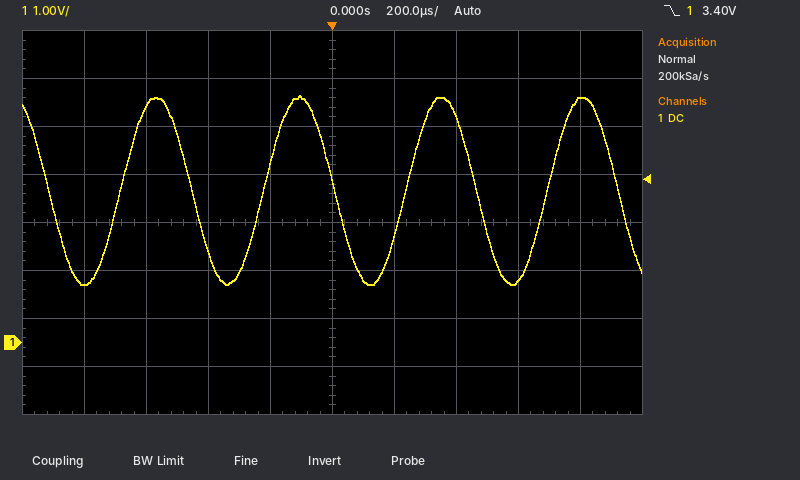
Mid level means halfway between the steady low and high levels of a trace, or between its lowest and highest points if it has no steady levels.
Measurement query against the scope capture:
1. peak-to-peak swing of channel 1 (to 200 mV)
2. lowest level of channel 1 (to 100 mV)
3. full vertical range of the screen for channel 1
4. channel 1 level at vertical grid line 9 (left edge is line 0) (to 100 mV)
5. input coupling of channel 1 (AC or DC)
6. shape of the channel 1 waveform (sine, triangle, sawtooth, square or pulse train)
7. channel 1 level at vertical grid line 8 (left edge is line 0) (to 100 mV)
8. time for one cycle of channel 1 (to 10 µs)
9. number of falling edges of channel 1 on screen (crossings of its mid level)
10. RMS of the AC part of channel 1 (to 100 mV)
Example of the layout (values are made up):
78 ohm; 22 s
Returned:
4.0 V; 1.2 V; 8 V; 5.1 V; DC; sine; 1.3 V; 460 µs; 5; 1.4 V
